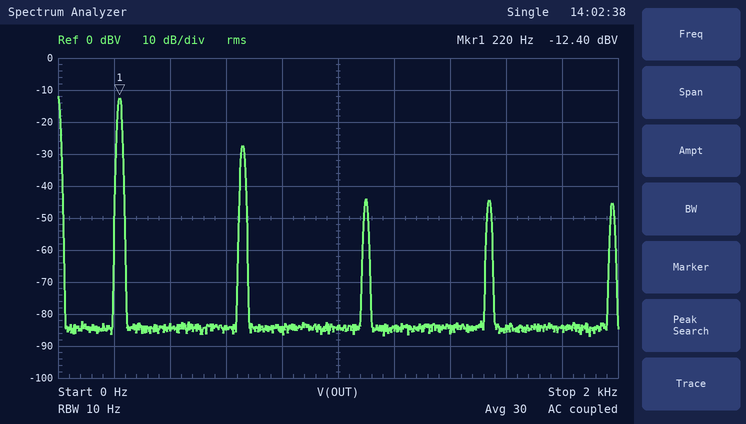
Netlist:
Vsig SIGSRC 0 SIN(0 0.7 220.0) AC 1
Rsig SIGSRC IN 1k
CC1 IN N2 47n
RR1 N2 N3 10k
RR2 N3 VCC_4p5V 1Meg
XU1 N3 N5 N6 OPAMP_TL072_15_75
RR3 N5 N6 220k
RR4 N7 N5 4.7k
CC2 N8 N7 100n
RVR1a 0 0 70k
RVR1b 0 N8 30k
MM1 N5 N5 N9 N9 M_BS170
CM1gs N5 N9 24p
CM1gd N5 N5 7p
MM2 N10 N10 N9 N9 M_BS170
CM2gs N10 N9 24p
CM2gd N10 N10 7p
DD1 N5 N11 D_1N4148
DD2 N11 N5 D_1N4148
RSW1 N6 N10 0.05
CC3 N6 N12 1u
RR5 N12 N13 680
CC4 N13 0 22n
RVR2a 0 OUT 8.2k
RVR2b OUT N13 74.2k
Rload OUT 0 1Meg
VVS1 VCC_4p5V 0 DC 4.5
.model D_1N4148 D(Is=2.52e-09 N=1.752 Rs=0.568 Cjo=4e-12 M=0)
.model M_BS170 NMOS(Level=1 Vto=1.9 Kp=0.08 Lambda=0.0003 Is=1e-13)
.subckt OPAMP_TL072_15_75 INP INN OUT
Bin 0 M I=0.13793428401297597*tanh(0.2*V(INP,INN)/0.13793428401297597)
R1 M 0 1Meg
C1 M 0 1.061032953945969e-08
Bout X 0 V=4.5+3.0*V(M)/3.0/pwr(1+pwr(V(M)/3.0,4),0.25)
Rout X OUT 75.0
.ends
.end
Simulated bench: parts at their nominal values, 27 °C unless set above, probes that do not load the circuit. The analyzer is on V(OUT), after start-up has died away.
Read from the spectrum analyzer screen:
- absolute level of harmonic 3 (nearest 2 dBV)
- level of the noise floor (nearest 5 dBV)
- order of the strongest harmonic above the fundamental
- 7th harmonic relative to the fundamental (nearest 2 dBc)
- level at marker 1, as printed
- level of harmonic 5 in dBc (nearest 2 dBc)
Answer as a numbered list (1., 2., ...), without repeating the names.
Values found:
1. -28 dBV
2. -85 dBV
3. 3
4. -32 dBc
5. -12.40 dBV
6. -32 dBc
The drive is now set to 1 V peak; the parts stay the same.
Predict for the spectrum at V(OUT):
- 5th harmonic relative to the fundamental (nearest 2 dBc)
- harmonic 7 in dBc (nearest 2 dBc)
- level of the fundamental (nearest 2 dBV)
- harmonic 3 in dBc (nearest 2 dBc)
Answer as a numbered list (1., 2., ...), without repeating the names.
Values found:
1. -14 dBc
2. -18 dBc
3. -12 dBV
4. -10 dBc
